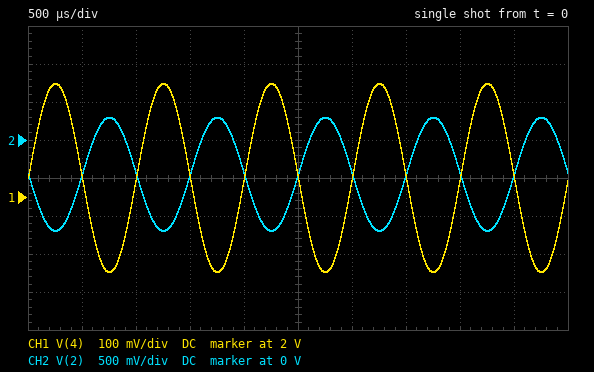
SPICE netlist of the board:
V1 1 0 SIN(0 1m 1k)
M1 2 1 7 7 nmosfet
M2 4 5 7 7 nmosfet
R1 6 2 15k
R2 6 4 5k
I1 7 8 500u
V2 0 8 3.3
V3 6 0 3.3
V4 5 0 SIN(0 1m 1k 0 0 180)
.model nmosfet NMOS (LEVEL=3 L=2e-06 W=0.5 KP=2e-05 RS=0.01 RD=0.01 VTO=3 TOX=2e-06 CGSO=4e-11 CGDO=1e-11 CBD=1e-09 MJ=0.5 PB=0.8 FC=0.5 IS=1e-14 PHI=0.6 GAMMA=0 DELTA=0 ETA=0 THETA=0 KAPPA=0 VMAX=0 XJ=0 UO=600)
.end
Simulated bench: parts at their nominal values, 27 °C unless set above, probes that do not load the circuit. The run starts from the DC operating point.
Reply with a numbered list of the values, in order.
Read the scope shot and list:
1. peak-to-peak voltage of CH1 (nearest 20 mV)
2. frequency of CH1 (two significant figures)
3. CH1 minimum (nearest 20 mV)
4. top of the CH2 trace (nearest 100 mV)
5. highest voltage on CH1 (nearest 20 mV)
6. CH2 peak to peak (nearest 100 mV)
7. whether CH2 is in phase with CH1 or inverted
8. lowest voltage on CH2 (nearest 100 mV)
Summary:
1. 500 mV
2. 1.0 kHz
3. 1.80 V
4. 300 mV
5. 2.30 V
6. 1.5 V
7. inverted
8. -1.2 V
